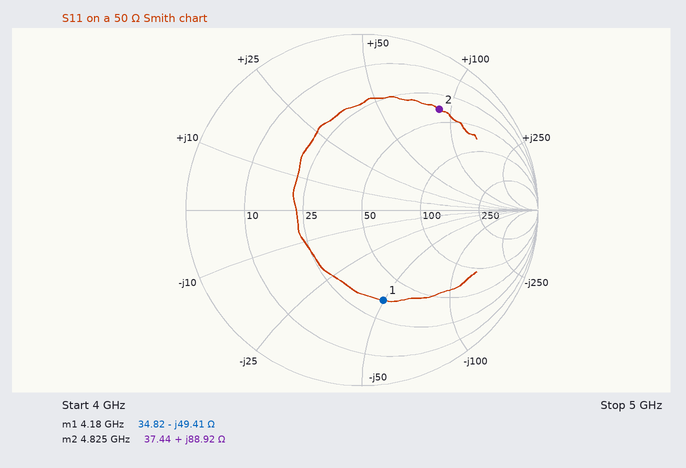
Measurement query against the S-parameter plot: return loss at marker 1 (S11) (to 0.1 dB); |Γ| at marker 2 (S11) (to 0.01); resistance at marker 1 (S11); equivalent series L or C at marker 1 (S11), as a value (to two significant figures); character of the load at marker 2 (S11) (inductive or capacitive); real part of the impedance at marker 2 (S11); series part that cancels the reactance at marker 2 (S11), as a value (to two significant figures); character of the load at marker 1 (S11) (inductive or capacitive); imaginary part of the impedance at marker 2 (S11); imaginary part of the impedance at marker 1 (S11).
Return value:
5.6 dB
0.72
34.82 Ω
770 fF
inductive
37.44 Ω
370 fF
capacitive
+88.92 Ω
-49.41 Ω
